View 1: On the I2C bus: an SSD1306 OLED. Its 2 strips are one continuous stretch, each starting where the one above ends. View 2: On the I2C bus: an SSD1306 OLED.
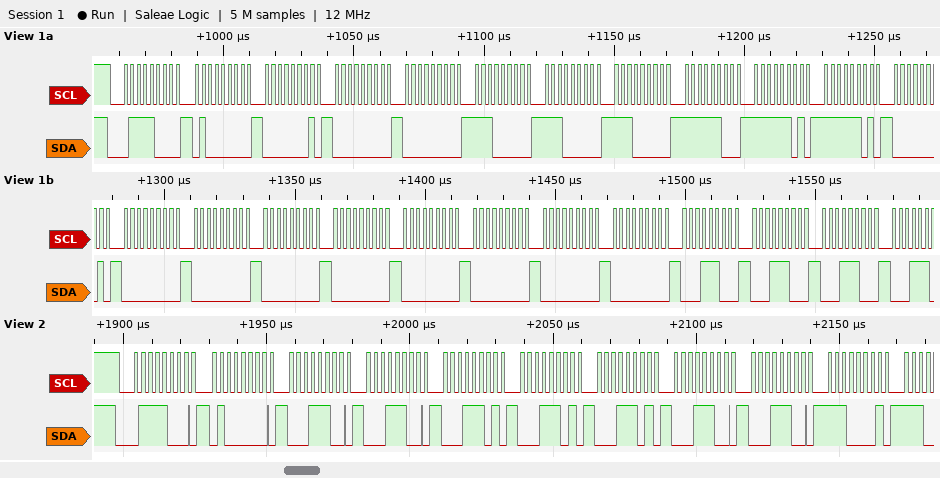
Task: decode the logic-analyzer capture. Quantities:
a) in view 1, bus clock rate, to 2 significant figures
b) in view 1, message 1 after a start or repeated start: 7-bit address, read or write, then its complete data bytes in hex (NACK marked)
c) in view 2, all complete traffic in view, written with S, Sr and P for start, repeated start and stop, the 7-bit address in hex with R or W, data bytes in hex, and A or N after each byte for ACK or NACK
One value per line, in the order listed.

400 kHz
0x3C write: 40 01 00 00 E0 E0 E0 FC FD FD 01 00 00 00 00 00 00 00 00 1C 1C 1C
S 3CW A 40 A 1C A 1C A 1D A 1D A 1D A 1C A 1C A E1 A
